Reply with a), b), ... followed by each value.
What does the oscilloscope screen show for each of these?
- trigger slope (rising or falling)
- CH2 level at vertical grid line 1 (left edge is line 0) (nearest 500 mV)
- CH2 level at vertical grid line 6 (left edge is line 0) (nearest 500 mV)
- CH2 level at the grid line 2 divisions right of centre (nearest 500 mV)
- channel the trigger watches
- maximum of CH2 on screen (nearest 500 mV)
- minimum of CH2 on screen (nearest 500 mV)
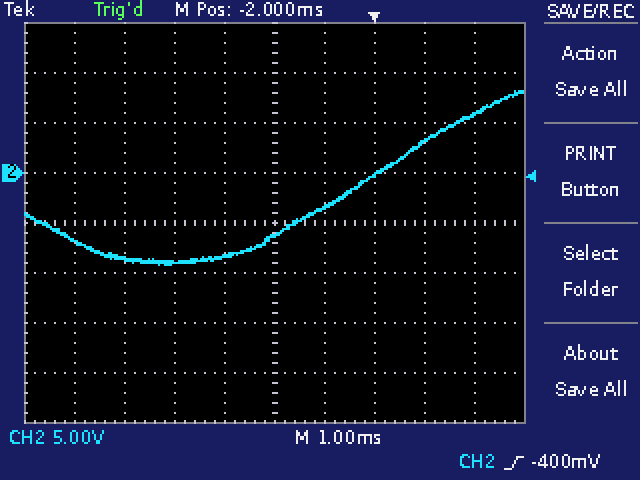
a) rising
b) -7.0 V
c) -3.5 V
d) 0.0 V
e) CH2
f) 8.0 V
g) -9.0 V
